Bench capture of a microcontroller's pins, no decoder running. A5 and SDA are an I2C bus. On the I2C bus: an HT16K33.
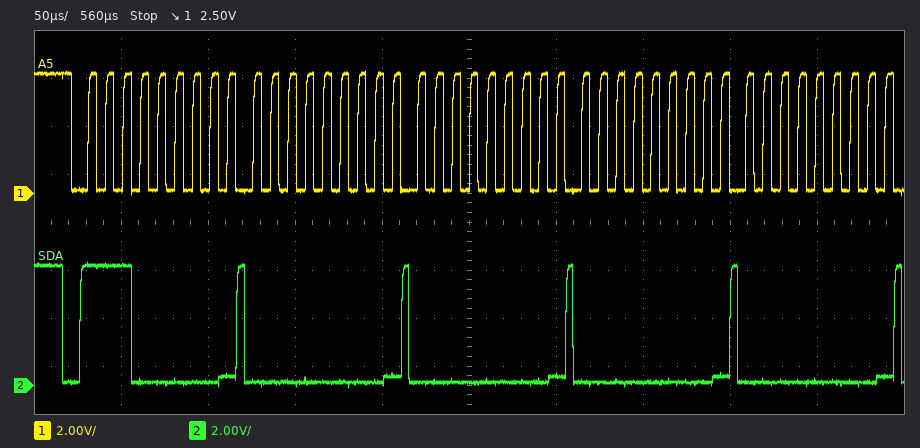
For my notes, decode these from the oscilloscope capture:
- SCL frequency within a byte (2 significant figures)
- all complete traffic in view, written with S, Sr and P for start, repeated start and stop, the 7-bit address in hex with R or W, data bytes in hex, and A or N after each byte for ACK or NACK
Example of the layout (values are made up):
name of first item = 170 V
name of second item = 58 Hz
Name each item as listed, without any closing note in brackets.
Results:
SCL frequency within a byte = 100 kHz
all complete traffic in view, written with S, Sr and P for start, repeated start and stop, the 7-bit address in hex with R or W, data bytes in hex, and A or N after each byte for ACK or NACK = S 70W A 00 A 00 A 00 A 00 A
